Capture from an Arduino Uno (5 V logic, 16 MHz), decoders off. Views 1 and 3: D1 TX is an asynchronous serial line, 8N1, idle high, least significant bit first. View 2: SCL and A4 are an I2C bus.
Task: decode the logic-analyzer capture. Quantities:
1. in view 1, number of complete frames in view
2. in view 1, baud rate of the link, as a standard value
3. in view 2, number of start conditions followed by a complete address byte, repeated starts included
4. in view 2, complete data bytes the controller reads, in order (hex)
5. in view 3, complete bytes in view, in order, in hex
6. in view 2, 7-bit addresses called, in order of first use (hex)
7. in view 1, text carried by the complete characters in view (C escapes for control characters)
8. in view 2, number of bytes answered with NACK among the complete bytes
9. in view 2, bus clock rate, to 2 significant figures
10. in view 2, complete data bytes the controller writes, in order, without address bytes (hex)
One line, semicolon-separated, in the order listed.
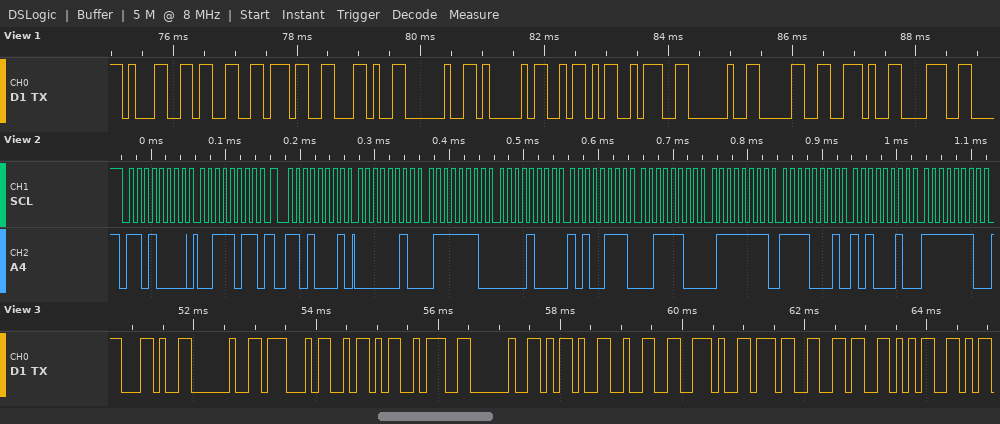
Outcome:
12; 9600 baud; 2; 02 7E 08 A7 3C 7F F1 A2 FE; 2C 20 47 5A 3A 20 2D 32 2E 37 36 35; 0x68; "137, AZ: 0.8"; 0; 100 kHz; 3B
